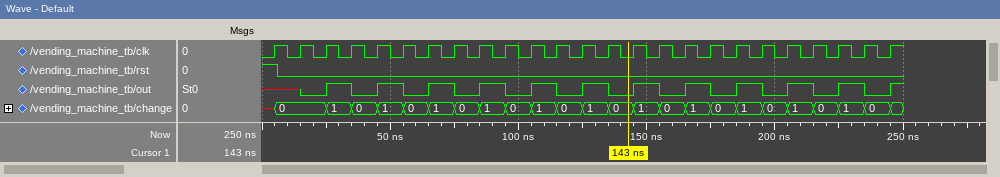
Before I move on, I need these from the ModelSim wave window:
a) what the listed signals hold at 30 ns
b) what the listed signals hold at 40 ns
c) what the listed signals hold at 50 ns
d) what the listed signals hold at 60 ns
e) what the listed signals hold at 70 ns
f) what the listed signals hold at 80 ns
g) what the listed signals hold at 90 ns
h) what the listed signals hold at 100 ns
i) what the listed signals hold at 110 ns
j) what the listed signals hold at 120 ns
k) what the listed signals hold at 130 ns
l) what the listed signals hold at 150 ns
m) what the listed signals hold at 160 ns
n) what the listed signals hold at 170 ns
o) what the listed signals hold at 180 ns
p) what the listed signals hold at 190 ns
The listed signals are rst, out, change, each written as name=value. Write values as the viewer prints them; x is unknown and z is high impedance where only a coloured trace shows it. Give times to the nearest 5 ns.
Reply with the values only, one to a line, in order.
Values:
rst=0, out=1, change=1
rst=0, out=0, change=0
rst=0, out=1, change=1
rst=0, out=0, change=0
rst=0, out=1, change=1
rst=0, out=0, change=0
rst=0, out=1, change=1
rst=0, out=0, change=0
rst=0, out=1, change=1
rst=0, out=0, change=0
rst=0, out=1, change=1
rst=0, out=1, change=1
rst=0, out=0, change=0
rst=0, out=1, change=1
rst=0, out=0, change=0
rst=0, out=1, change=1
